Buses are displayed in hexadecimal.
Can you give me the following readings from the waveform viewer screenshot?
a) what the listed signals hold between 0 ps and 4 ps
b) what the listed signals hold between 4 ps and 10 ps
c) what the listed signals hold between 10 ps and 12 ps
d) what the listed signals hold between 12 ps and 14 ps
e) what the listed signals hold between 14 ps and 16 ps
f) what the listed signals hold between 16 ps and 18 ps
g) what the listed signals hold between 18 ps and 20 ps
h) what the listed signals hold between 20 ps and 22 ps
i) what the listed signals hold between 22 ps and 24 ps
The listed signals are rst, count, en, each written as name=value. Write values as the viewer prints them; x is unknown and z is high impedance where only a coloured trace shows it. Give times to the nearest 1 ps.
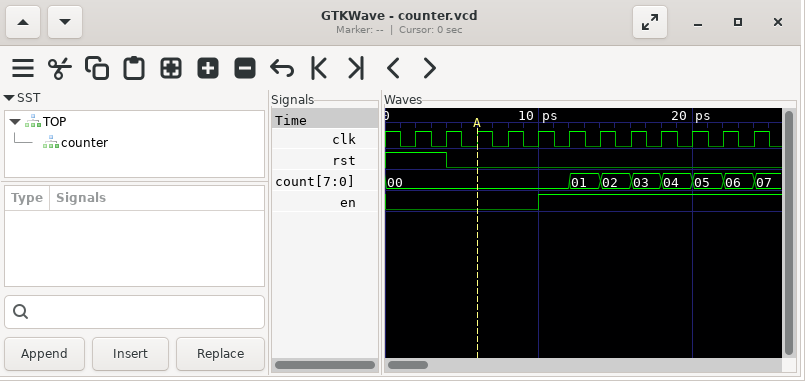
rst=1, count=00, en=0
rst=0, count=00, en=0
rst=0, count=00, en=1
rst=0, count=01, en=1
rst=0, count=02, en=1
rst=0, count=03, en=1
rst=0, count=04, en=1
rst=0, count=05, en=1
rst=0, count=06, en=1
